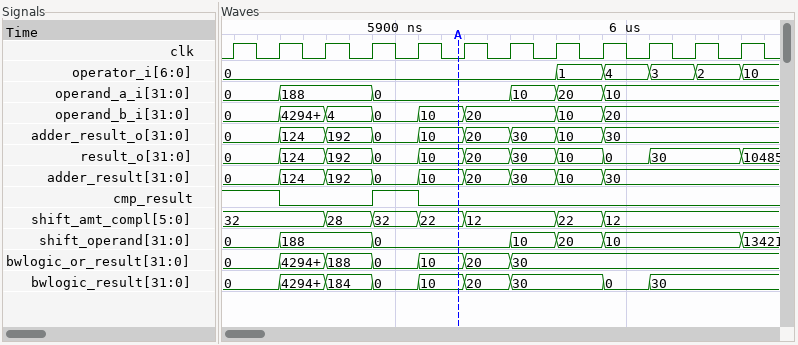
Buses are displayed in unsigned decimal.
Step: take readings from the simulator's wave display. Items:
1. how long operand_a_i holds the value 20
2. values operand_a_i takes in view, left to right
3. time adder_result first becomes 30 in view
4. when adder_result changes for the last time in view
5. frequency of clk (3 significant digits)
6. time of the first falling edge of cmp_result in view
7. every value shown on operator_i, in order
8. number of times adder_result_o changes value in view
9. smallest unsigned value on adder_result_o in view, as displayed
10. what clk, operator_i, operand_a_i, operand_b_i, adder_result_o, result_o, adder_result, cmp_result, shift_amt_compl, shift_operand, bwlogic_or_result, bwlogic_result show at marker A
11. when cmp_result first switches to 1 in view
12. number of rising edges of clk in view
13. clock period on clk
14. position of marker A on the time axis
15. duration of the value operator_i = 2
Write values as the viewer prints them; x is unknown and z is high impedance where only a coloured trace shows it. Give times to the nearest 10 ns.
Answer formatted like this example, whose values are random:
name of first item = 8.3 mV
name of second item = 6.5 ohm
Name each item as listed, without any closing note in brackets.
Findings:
how long operand_a_i holds the value 20 = 20 ns
values operand_a_i takes in view, left to right = 0, 188, 0, 10, 20, 10
time adder_result first becomes 30 in view = 5950 ns
when adder_result changes for the last time in view = 5990 ns
frequency of clk = 50.0 MHz
time of the first falling edge of cmp_result in view = 5850 ns
every value shown on operator_i, in order = 0, 1, 4, 3, 2, 10
number of times adder_result_o changes value in view = 8
smallest unsigned value on adder_result_o in view, as displayed = 0
what clk, operator_i, operand_a_i, operand_b_i, adder_result_o, result_o, adder_result, cmp_result, shift_amt_compl, shift_operand, bwlogic_or_result, bwlogic_result show at marker A = clk=0, operator_i=0, operand_a_i=0, operand_b_i=10, adder_result_o=10, result_o=10, adder_result=10, cmp_result=0, shift_amt_compl=22, shift_operand=0, bwlogic_or_result=10, bwlogic_result=10
when cmp_result first switches to 1 in view = 5890 ns
number of rising edges of clk in view = 12
clock period on clk = 20 ns
position of marker A on the time axis = 5930 ns
duration of the value operator_i = 2 = 20 ns
